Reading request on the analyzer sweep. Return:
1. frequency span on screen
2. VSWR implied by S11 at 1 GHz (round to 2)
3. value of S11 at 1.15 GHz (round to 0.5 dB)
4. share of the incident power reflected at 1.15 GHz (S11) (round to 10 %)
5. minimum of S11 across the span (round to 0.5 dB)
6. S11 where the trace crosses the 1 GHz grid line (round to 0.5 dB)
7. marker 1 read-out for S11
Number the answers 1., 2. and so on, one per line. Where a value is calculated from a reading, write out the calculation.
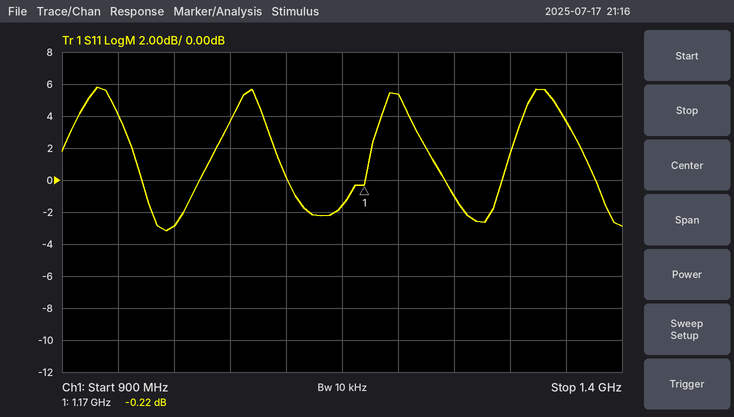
1. 500 MHz
2. |Γ| = 10^(-3/20) = 0.7079; VSWR = (1 + 0.7079)/(1 − 0.7079) ≈ 6
3. -1.5 dB
4. 10^(-1.5/10) ≈ 70.8 %, so 70 % to the nearest 10 %
5. -3.0 dB
6. -3.0 dB
7. -0.22 dB
